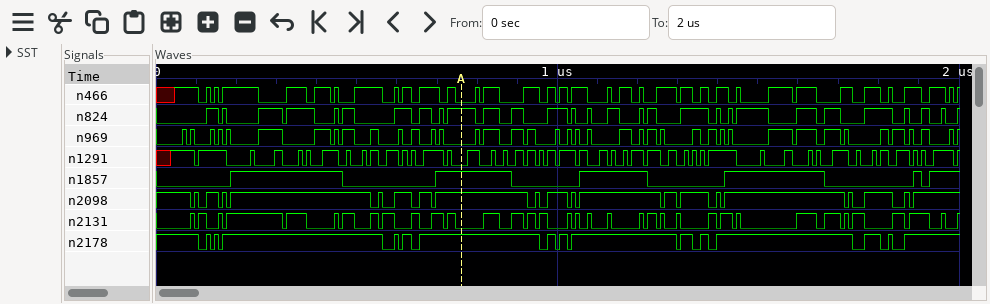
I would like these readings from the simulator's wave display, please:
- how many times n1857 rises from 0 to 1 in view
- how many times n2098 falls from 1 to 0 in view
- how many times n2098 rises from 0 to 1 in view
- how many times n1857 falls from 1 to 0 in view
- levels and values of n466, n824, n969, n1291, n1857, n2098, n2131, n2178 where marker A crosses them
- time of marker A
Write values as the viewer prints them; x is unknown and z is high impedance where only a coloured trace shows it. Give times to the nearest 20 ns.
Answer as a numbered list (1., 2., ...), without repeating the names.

1. 6
2. 20
3. 20
4. 5
5. n466=0, n824=1, n969=0, n1291=0, n1857=1, n2098=1, n2131=0, n2178=1
6. 760 ns
